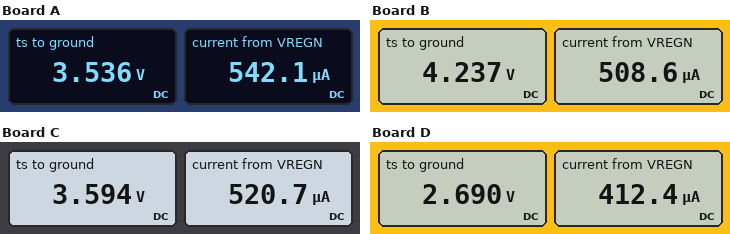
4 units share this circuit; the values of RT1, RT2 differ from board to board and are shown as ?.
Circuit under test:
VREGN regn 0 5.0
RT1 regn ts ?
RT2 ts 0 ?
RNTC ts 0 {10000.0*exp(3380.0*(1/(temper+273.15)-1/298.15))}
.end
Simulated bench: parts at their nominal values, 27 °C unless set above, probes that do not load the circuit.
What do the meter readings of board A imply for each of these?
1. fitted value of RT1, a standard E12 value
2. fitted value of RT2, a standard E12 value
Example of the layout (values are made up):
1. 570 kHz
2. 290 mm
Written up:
1. 2.7 kΩ
2. 22 kΩ
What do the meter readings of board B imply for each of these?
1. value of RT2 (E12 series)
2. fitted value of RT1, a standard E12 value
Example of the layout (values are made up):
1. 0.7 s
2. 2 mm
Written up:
1. 82 kΩ
2. 1.5 kΩ
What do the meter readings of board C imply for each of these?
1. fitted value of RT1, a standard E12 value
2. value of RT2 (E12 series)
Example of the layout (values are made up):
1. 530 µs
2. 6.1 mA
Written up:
1. 2.7 kΩ
2. 27 kΩ
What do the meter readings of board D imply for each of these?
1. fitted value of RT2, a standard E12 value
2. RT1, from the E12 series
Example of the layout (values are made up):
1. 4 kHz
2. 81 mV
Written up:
1. 22 kΩ
2. 5.6 kΩ
